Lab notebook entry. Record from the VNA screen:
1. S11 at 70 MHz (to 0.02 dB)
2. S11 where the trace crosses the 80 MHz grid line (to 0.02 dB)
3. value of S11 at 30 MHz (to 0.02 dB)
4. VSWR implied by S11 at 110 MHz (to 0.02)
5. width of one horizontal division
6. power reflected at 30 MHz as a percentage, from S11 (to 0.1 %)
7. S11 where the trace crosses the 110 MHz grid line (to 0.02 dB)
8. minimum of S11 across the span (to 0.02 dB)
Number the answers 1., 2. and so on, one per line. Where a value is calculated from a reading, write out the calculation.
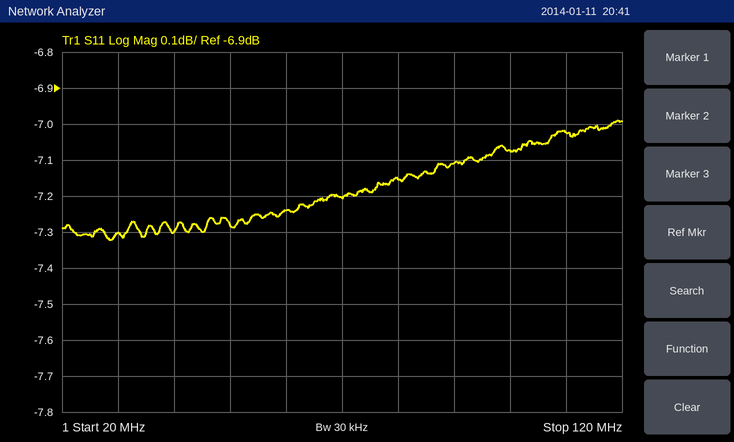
1. -7.20 dB
2. -7.16 dB
3. -7.30 dB
4. |Γ| = 10^(-7.02/20) = 0.4457; VSWR = (1 + 0.4457)/(1 − 0.4457) ≈ 2.61, so 2.60 to the nearest 0.02
5. 10 MHz
6. 10^(-7.3/10) ≈ 18.6 %
7. -7.02 dB
8. -7.32 dB
